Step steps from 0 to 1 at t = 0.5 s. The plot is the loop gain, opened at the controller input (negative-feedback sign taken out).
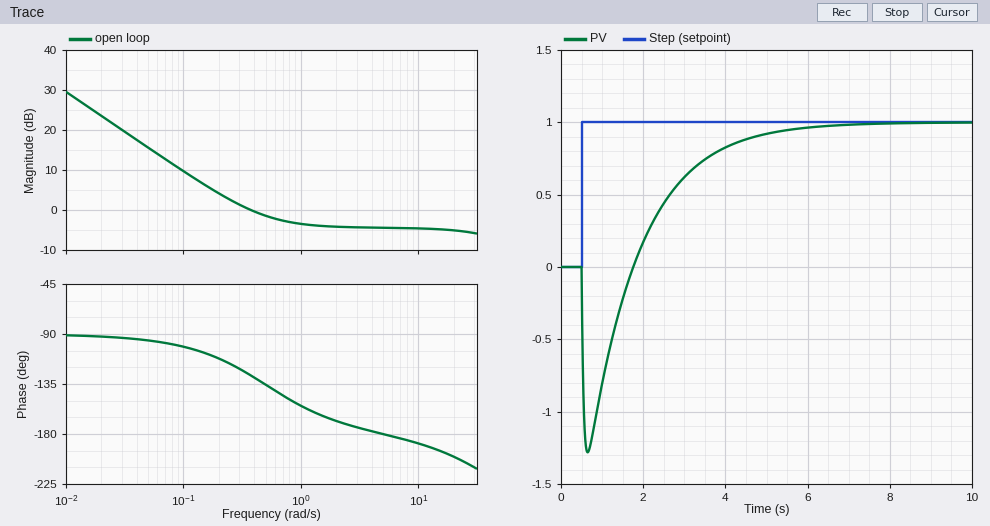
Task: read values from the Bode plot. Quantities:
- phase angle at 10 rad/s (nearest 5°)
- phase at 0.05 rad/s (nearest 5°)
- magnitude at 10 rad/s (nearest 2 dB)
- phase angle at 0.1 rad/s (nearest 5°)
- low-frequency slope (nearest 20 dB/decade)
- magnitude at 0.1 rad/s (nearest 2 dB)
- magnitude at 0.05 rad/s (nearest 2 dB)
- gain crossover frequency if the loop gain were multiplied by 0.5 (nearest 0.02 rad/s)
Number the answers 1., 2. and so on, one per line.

1. -190°
2. -95°
3. -4 dB
4. -100°
5. -20 dB/decade
6. 10 dB
7. 16 dB
8. 0.16 rad/s
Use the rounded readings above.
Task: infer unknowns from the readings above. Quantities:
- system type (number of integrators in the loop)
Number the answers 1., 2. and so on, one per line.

1. 1
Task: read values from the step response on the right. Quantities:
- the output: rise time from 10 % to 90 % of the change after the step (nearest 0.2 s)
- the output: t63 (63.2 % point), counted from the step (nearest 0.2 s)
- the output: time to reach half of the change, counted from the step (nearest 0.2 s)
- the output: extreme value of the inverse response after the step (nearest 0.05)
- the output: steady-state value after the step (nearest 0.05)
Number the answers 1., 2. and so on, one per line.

1. 2.8 s
2. 2.6 s
3. 2.2 s
4. -1.30
5. 1.00
